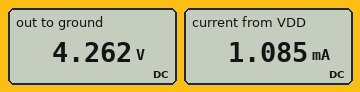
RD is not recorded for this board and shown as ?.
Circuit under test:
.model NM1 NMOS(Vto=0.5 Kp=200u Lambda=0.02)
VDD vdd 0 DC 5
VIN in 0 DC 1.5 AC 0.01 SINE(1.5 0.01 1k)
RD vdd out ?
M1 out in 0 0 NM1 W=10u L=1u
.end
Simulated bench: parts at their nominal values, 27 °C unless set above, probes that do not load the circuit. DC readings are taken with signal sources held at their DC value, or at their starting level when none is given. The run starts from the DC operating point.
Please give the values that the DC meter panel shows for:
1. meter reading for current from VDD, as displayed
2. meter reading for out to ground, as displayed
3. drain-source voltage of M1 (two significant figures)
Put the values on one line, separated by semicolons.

1.085 mA; 4.262 V; 4.3 V
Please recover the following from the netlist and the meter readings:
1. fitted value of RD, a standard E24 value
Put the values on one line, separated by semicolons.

680 Ω
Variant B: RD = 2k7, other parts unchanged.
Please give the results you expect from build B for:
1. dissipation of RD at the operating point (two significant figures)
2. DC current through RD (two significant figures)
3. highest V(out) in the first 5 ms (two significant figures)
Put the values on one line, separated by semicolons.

2.9 mW; 1.0 mA; 2.2 V
